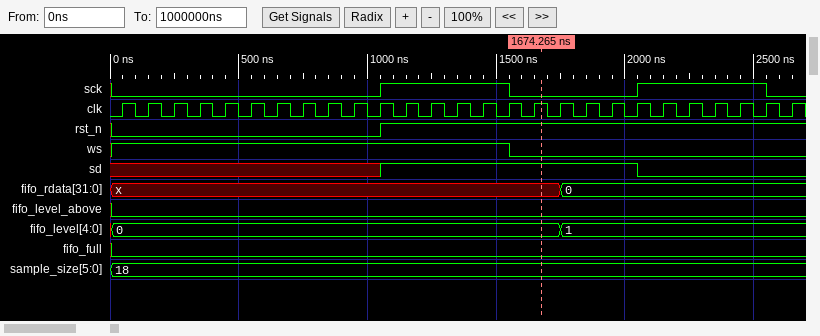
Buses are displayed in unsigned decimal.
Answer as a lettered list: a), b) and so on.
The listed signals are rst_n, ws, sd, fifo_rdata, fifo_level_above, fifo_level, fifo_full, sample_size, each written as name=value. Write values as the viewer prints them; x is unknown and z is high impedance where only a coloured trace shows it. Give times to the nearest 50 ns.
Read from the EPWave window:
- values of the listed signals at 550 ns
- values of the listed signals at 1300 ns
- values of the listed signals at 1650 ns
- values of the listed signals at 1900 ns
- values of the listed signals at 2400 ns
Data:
a) rst_n=0, ws=1, sd=x, fifo_rdata=x, fifo_level_above=0, fifo_level=0, fifo_full=0, sample_size=18
b) rst_n=1, ws=1, sd=1, fifo_rdata=x, fifo_level_above=0, fifo_level=0, fifo_full=0, sample_size=18
c) rst_n=1, ws=0, sd=1, fifo_rdata=x, fifo_level_above=0, fifo_level=0, fifo_full=0, sample_size=18
d) rst_n=1, ws=0, sd=1, fifo_rdata=0, fifo_level_above=0, fifo_level=1, fifo_full=0, sample_size=18
e) rst_n=1, ws=0, sd=0, fifo_rdata=0, fifo_level_above=0, fifo_level=1, fifo_full=0, sample_size=18
